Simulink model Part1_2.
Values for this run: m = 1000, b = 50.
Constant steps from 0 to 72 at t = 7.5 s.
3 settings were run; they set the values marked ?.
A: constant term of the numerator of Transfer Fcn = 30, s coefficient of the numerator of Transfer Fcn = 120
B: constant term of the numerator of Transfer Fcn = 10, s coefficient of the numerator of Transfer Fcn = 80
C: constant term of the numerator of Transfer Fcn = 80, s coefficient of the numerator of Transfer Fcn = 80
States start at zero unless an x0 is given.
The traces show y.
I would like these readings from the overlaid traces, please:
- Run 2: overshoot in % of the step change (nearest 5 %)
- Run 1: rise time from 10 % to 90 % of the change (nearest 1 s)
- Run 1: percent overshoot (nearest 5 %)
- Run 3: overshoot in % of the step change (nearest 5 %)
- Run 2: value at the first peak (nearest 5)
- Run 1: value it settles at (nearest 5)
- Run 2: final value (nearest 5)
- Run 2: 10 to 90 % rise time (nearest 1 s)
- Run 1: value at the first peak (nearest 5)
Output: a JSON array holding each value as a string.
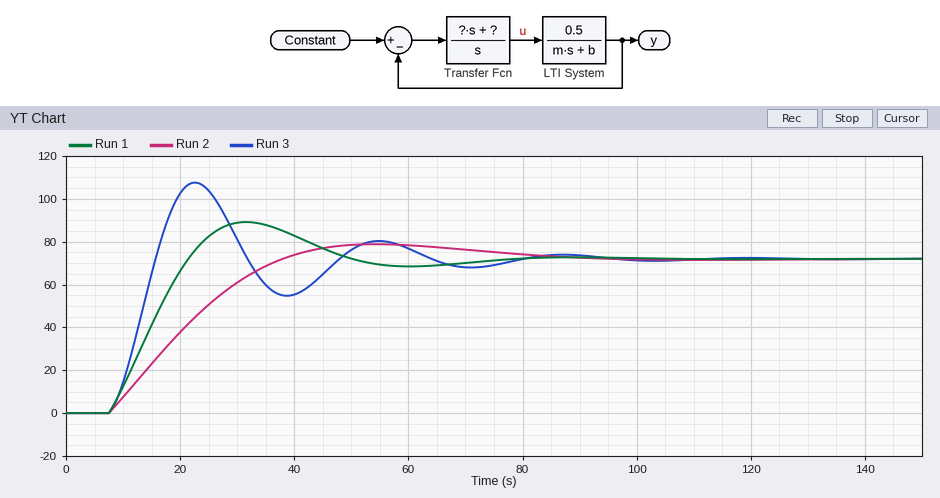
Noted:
["10 %", "11 s", "25 %", "50 %", "80", "70", "70", "22 s", "90"]
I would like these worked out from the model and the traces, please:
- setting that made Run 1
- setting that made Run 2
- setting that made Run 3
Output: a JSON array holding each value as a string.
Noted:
["A", "B", "C"]
